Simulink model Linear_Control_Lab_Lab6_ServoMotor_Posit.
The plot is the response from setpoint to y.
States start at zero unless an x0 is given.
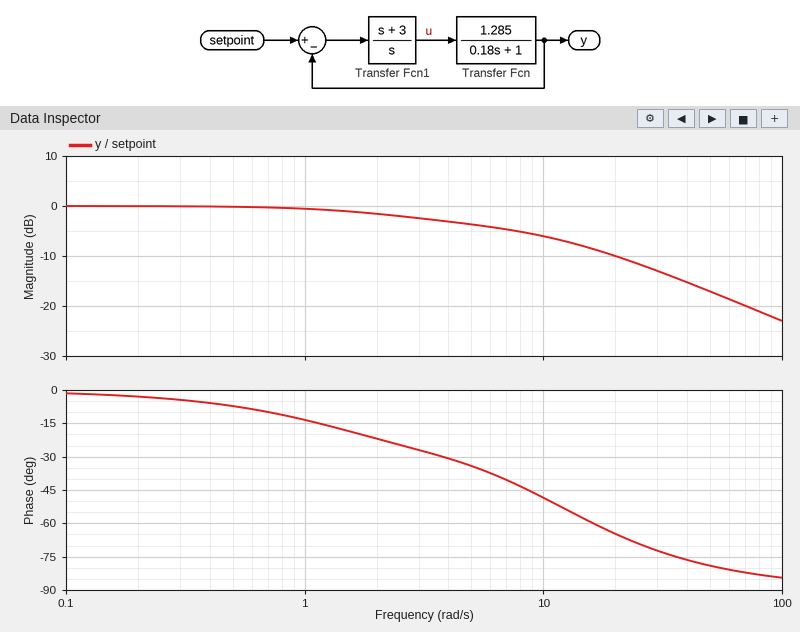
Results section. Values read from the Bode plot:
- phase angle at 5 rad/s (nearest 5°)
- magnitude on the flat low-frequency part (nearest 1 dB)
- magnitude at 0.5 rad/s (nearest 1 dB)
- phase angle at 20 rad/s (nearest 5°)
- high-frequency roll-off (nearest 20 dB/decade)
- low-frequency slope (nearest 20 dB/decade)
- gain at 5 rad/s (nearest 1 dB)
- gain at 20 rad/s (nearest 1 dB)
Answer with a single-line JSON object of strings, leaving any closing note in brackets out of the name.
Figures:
{"phase angle at 5 rad/s": "-35°", "magnitude on the flat low-frequency part": "0 dB", "magnitude at 0.5 rad/s": "0 dB", "phase angle at 20 rad/s": "-65°", "high-frequency roll-off": "-20 dB/decade", "low-frequency slope": "0 dB/decade", "gain at 5 rad/s": "-4 dB", "gain at 20 rad/s": "-10 dB"}
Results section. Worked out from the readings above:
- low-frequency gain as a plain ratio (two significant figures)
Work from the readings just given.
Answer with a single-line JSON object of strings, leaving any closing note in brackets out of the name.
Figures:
{"low-frequency gain as a plain ratio": "1.0"}
